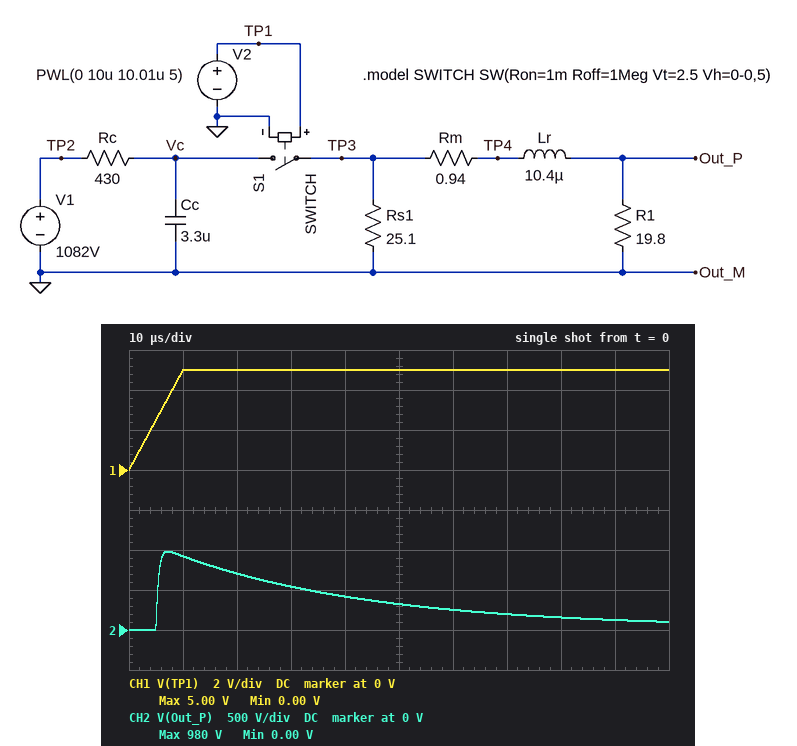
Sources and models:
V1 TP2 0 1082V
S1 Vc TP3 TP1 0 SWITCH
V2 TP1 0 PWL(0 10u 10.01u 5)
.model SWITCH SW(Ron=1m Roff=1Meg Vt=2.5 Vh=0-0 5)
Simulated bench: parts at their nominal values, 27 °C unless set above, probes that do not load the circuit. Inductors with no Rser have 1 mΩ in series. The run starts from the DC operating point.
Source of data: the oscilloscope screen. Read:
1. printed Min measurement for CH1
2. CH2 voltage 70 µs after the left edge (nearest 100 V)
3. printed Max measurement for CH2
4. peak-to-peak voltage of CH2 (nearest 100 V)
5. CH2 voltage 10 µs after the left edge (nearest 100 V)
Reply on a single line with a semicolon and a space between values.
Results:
0.00 V; 200 V; 980 V; 1.0 kV; 900 V
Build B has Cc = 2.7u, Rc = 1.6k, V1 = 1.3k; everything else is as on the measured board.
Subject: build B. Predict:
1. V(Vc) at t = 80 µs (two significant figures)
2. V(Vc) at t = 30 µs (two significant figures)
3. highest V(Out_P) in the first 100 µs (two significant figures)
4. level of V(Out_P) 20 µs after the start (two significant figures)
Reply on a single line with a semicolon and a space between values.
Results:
120 V; 580 V; 1.2 kV; 780 V
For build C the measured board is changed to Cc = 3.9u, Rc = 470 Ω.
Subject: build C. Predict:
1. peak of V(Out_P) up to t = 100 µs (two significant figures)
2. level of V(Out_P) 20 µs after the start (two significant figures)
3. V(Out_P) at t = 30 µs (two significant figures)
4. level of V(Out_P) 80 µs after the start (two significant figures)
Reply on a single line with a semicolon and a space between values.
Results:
990 V; 750 V; 600 V; 200 V
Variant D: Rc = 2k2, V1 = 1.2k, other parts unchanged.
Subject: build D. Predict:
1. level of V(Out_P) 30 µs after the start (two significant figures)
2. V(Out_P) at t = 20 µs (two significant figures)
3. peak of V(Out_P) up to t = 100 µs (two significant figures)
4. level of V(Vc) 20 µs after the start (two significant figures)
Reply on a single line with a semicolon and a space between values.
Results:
600 V; 780 V; 1.1 kV; 810 V
